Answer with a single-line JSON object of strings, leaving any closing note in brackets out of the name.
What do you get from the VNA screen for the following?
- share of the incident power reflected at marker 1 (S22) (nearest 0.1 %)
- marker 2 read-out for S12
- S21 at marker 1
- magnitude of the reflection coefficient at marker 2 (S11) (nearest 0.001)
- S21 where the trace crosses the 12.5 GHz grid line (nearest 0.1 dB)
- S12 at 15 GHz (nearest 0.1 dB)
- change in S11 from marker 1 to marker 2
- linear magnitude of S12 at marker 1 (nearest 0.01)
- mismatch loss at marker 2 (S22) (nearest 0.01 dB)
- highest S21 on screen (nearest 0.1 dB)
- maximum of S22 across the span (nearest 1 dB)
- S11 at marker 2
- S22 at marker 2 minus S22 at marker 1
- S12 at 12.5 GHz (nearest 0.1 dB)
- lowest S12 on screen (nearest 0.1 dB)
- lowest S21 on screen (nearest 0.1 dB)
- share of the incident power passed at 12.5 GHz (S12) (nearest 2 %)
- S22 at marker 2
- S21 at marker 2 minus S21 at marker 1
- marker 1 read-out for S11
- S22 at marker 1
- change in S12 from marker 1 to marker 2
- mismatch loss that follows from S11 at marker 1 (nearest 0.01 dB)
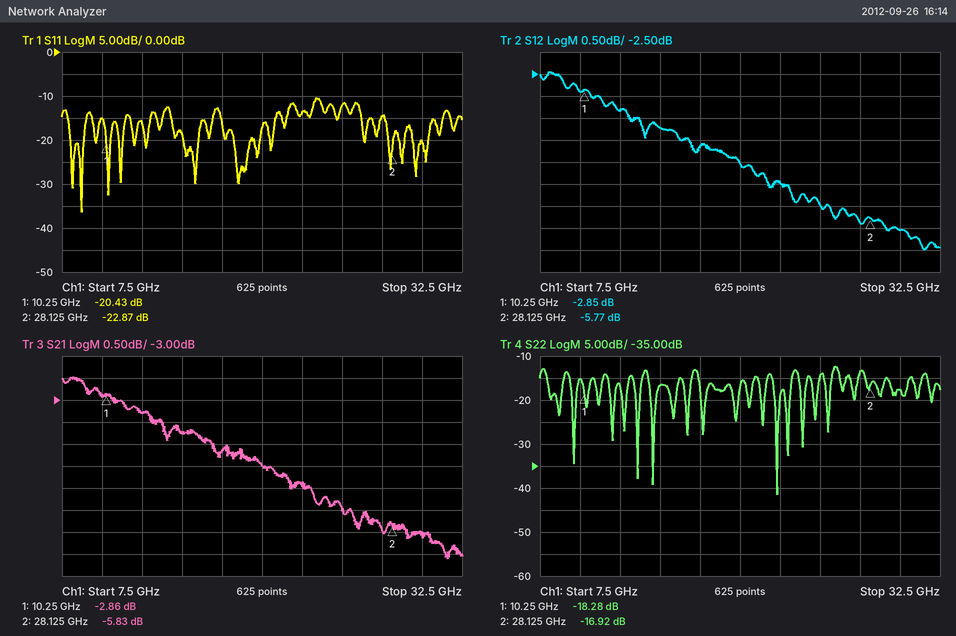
{"share of the incident power reflected at marker 1 (S22)": "1.5 %", "marker 2 read-out for S12": "-5.77 dB", "S21 at marker 1": "-2.86 dB", "magnitude of the reflection coefficient at marker 2 (S11)": "0.072", "S21 where the trace crosses the 12.5 GHz grid line": "-3.3 dB", "S12 at 15 GHz": "-3.7 dB", "change in S11 from marker 1 to marker 2": "-2.44 dB", "linear magnitude of S12 at marker 1": "0.72", "mismatch loss at marker 2 (S22)": "0.09 dB", "highest S21 on screen": "-2.5 dB", "maximum of S22 across the span": "-12 dB", "S11 at marker 2": "-22.87 dB", "S22 at marker 2 minus S22 at marker 1": "1.36 dB", "S12 at 12.5 GHz": "-3.3 dB", "lowest S12 on screen": "-6.5 dB", "lowest S21 on screen": "-6.6 dB", "share of the incident power passed at 12.5 GHz (S12)": "46 %", "S22 at marker 2": "-16.92 dB", "S21 at marker 2 minus S21 at marker 1": "-2.97 dB", "marker 1 read-out for S11": "-20.43 dB", "S22 at marker 1": "-18.28 dB", "change in S12 from marker 1 to marker 2": "-2.92 dB", "mismatch loss that follows from S11 at marker 1": "0.04 dB"}
